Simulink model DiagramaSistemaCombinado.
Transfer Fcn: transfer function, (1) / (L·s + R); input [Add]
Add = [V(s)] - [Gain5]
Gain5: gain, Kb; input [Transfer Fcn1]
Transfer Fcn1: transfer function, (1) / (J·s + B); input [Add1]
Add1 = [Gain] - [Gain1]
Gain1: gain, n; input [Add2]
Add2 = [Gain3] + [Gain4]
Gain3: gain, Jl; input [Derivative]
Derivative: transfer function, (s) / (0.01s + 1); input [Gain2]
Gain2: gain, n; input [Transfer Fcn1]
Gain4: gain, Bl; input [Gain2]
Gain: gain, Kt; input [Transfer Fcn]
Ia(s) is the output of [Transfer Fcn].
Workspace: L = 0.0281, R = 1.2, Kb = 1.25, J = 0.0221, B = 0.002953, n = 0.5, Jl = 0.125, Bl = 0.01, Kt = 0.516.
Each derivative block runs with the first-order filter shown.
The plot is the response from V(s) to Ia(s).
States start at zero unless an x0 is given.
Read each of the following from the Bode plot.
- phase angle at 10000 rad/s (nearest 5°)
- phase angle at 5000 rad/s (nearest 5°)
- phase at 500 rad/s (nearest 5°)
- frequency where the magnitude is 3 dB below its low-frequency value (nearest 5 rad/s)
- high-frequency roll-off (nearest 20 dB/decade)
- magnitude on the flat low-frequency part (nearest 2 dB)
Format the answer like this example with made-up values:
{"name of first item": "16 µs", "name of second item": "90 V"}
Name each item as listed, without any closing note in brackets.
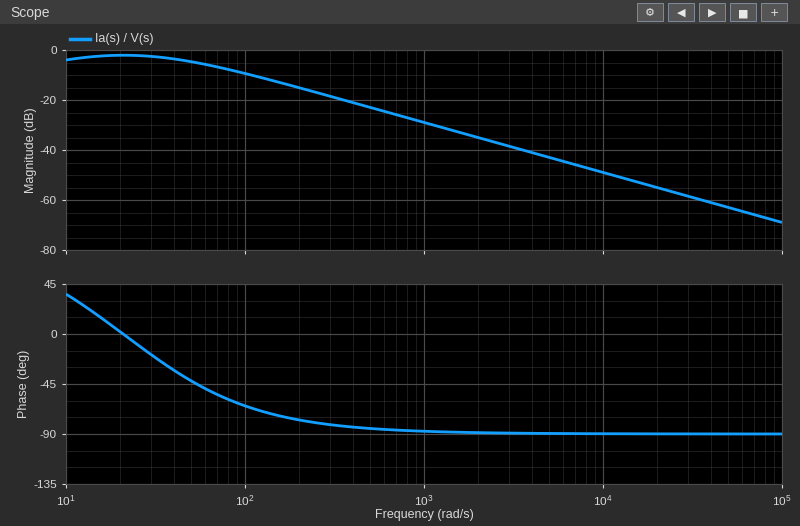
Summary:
{"phase angle at 10000 rad/s": "-90°", "phase angle at 5000 rad/s": "-90°", "phase at 500 rad/s": "-85°", "frequency where the magnitude is 3 dB below its low-frequency value": "60 rad/s", "high-frequency roll-off": "-20 dB/decade", "magnitude on the flat low-frequency part": "-2 dB"}
